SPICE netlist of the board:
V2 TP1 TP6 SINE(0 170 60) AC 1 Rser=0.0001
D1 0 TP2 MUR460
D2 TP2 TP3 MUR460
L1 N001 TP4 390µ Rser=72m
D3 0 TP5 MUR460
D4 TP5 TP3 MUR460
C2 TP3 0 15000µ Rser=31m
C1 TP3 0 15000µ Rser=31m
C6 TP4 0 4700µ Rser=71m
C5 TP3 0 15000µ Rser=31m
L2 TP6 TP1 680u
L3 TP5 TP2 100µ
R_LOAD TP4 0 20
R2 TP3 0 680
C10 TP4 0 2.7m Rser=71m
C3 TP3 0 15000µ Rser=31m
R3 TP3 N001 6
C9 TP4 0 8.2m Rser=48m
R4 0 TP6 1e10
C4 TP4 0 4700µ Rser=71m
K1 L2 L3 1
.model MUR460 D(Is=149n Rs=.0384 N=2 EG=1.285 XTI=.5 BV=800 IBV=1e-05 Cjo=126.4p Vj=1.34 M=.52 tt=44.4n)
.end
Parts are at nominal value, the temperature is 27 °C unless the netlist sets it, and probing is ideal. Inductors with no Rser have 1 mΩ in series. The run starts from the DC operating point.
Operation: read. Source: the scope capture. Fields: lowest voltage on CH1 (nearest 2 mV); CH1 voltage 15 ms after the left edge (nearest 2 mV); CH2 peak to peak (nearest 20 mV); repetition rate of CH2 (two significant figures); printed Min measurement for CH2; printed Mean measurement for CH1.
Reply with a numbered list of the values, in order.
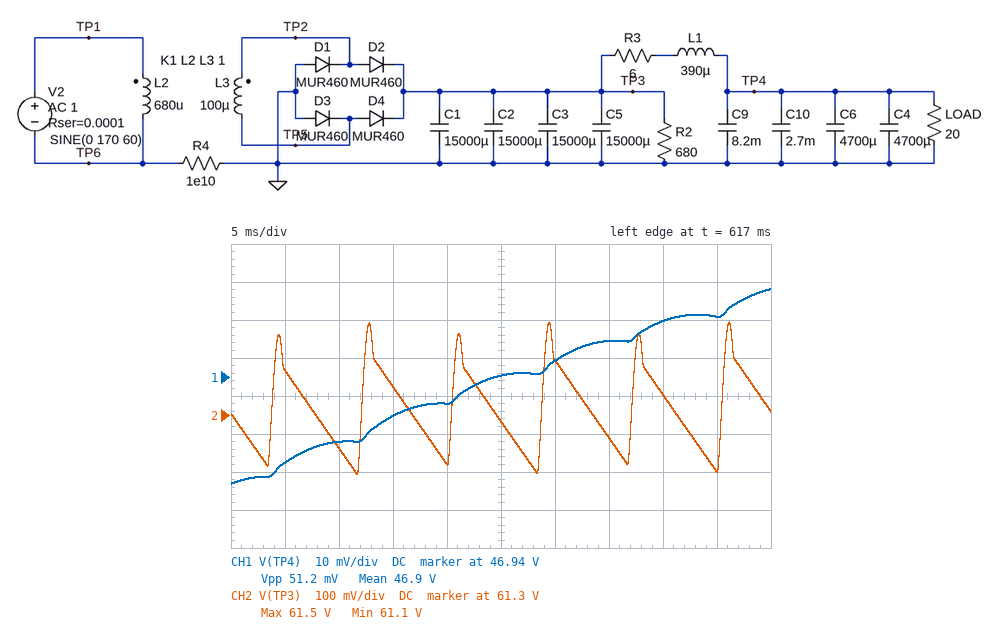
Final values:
1. 46.912 V
2. 46.930 V
3. 400 mV
4. 120 Hz
5. 61.1 V
6. 46.9 V
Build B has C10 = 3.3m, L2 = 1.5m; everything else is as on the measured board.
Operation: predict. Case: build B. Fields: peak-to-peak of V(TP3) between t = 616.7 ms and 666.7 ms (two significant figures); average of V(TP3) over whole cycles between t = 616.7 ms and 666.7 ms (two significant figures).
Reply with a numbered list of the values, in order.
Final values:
1. 260 mV
2. 41 V
